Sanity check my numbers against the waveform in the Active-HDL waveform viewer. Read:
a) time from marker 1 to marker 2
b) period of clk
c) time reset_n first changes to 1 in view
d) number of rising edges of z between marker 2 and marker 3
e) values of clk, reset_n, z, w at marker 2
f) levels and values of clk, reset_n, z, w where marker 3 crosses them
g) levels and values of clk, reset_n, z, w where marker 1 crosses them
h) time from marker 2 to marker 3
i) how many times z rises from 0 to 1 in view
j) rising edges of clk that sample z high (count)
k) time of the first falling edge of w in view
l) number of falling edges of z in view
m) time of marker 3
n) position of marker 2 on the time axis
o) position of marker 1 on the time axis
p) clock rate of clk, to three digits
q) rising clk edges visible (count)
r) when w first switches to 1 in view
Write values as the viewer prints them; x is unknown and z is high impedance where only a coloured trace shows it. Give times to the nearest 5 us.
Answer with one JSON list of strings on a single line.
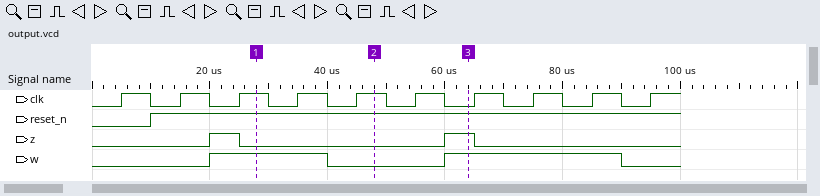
["20 us", "10 us", "10 us", "1", "clk=1, reset_n=1, z=0, w=0", "clk=0, reset_n=1, z=1, w=1", "clk=1, reset_n=1, z=0, w=1", "15 us", "2", "2", "40 us", "2", "65 us", "50 us", "30 us", "100 kHz", "10", "20 us"]
